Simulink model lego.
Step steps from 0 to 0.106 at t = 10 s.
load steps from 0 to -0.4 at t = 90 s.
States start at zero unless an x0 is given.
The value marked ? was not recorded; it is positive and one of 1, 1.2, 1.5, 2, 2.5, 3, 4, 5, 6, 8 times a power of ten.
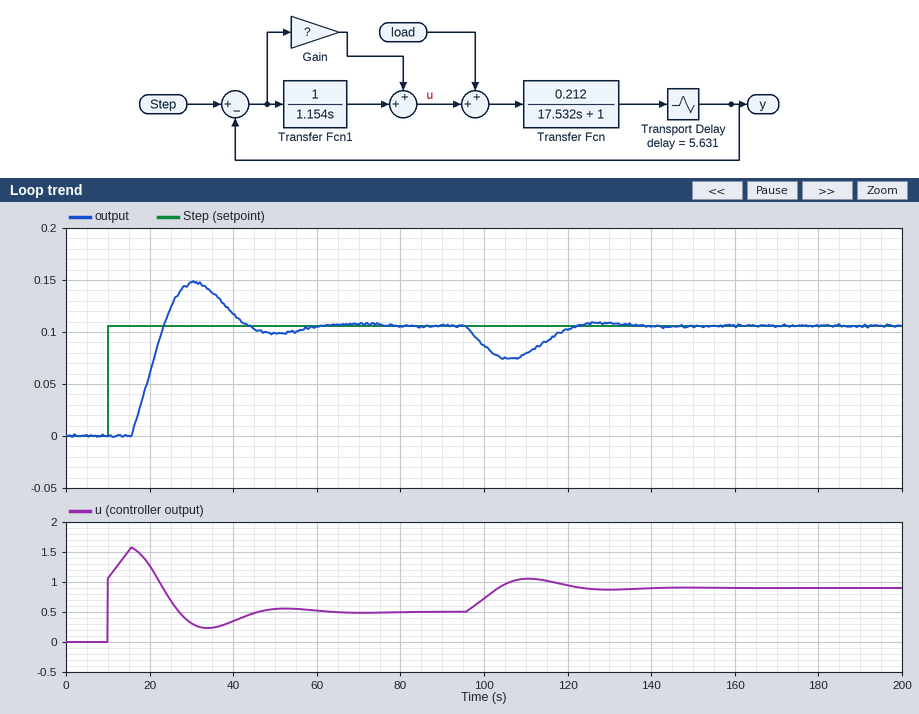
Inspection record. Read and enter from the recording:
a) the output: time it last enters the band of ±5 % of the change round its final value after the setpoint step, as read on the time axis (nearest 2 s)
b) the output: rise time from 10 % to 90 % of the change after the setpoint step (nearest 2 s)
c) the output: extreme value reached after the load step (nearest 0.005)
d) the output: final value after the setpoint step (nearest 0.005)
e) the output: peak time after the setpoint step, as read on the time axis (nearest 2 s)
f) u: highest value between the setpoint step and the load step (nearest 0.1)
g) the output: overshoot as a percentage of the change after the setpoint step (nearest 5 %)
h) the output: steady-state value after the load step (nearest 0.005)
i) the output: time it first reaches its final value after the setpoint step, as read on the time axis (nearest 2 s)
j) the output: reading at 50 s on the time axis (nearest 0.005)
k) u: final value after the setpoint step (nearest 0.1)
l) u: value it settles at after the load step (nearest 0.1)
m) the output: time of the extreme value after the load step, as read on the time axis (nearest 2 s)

54 s
6 s
0.075
0.105
30 s
1.6
40 %
0.105
24 s
0.100
0.5
0.9
106 s
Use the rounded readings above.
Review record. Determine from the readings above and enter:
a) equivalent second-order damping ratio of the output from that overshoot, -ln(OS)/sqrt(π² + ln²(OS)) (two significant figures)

0.28
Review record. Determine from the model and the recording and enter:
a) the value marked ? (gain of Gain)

10
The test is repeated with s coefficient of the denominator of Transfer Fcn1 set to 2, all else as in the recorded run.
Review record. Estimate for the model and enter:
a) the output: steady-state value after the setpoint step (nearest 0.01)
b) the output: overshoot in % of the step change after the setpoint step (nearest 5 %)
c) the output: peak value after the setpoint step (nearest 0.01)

0.11
15 %
0.12
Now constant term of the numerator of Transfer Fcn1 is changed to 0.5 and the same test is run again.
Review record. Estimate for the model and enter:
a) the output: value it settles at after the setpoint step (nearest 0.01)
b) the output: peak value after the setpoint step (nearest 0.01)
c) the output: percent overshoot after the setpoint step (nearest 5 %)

0.11
0.12
10 %
